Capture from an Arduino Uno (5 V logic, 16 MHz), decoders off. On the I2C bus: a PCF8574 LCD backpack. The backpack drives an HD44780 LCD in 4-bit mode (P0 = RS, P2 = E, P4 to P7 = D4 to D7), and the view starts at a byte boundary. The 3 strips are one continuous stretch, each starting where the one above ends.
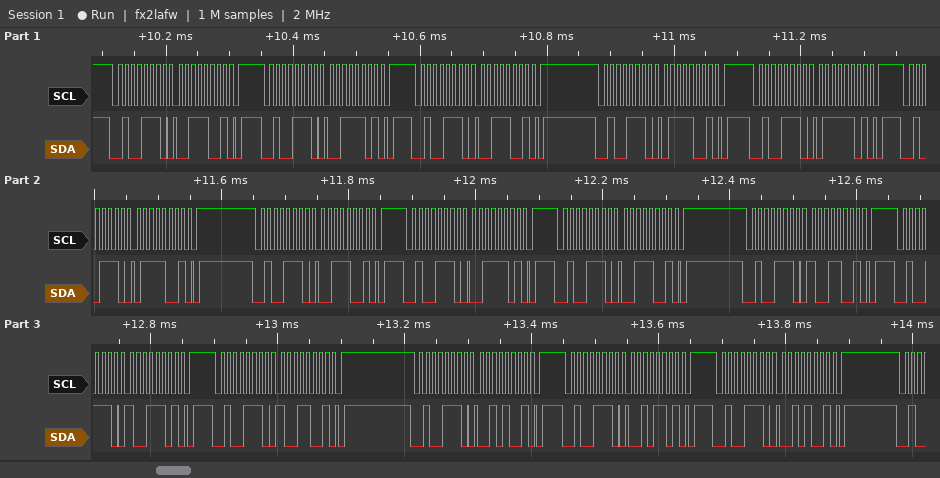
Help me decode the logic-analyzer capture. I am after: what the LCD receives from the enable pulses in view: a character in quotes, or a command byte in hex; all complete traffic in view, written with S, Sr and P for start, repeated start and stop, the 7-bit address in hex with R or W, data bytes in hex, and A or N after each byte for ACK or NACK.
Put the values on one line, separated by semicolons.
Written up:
'7' '9'; S 27W A 39 A P S 27W A 3D A P S 27W A 39 A P S 27W A 79 A P S 27W A 7D A P S 27W A 79 A P S 27W A 39 A P S 27W A 3D A P S 27W A 39 A P S 27W A 99 A P S 27W A 9D A P S 27W A 99 A P S 27W A 29 A P S 27W A 2D A P S 27W A 29 A P
